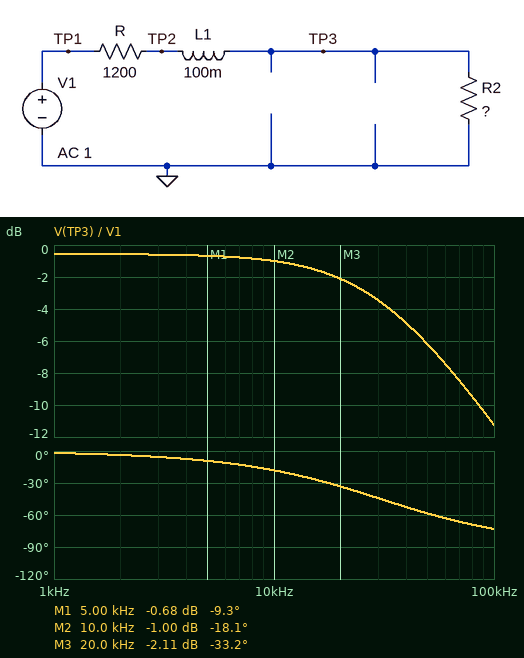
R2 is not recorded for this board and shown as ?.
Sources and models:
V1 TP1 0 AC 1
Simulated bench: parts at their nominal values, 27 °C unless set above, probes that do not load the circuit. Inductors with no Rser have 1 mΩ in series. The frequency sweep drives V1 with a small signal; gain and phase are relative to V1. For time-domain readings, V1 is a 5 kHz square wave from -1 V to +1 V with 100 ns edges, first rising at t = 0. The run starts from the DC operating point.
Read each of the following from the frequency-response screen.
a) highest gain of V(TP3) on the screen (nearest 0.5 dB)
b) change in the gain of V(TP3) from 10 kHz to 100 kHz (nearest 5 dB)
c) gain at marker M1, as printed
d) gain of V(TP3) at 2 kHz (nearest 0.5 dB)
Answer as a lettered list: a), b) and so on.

a) -0.5 dB
b) -10 dB
c) -0.68 dB
d) -0.5 dB
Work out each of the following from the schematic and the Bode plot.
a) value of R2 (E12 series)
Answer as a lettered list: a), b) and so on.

a) 18 kΩ
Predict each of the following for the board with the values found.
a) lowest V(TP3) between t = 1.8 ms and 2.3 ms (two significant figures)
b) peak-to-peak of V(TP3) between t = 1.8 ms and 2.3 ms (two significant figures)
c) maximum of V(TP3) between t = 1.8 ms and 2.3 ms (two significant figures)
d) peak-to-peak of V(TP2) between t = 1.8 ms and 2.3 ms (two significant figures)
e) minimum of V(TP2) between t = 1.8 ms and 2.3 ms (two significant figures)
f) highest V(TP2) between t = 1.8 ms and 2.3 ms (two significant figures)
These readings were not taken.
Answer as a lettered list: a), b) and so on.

a) -940 mV
b) 1.9 V
c) 940 mV
d) 2.1 V
e) -1.1 V
f) 1.1 V
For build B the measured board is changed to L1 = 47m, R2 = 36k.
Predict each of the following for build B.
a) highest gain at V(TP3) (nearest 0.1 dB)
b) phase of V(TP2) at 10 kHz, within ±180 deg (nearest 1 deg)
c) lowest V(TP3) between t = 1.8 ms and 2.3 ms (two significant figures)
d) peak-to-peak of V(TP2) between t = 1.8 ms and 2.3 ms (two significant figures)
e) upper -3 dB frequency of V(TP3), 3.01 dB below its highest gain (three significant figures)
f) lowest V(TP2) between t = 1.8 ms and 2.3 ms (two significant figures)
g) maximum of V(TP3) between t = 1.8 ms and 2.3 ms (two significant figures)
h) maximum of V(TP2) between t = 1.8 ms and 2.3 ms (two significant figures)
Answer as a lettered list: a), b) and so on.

a) -0.3 dB
b) 0 deg
c) -970 mV
d) 2.1 V
e) 126 kHz
f) -1.0 V
g) 970 mV
h) 1.0 V
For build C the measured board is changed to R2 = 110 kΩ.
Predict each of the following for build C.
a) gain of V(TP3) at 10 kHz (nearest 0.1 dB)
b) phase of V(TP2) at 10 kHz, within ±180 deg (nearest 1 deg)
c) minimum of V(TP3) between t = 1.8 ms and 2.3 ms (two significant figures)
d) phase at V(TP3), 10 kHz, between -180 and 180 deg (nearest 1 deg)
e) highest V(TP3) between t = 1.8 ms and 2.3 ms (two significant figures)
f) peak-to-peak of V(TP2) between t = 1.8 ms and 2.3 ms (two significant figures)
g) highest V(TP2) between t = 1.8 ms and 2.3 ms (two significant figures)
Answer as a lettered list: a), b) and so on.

a) -0.1 dB
b) 0 deg
c) -990 mV
d) -3 deg
e) 990 mV
f) 2.0 V
g) 1.0 V
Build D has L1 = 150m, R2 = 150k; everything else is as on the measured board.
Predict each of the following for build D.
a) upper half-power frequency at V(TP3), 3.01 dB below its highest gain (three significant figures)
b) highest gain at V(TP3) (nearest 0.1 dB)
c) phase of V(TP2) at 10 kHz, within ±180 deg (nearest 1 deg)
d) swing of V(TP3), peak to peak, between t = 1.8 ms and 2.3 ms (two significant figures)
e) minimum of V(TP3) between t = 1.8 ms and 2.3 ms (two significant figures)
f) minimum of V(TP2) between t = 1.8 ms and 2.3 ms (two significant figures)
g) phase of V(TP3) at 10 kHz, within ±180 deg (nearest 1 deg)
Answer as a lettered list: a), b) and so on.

a) 160 kHz
b) -0.1 dB
c) 0 deg
d) 2.0 V
e) -990 mV
f) -1.0 V
g) -4 deg
